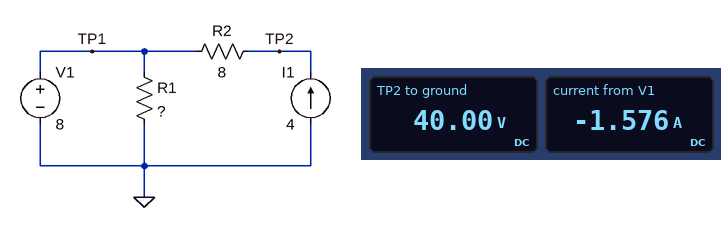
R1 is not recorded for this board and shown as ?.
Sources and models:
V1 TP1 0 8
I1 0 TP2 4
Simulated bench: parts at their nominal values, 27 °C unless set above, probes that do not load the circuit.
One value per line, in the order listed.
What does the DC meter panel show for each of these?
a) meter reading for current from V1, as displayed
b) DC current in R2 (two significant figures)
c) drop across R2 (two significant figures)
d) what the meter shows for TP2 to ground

-1.576 A
4.0 A
32 V
40.00 V
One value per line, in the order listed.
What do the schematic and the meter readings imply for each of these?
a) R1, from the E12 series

3.3 Ω
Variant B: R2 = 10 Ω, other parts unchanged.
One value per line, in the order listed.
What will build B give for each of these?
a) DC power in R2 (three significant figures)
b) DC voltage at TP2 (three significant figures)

160 W
48.0 V
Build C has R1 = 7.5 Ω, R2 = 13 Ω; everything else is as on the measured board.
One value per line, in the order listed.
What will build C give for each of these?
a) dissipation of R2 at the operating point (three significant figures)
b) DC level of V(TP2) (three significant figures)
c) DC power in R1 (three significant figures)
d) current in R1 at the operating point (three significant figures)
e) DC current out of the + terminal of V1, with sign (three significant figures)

208 W
60.0 V
8.53 W
1.07 A
-2.93 A
